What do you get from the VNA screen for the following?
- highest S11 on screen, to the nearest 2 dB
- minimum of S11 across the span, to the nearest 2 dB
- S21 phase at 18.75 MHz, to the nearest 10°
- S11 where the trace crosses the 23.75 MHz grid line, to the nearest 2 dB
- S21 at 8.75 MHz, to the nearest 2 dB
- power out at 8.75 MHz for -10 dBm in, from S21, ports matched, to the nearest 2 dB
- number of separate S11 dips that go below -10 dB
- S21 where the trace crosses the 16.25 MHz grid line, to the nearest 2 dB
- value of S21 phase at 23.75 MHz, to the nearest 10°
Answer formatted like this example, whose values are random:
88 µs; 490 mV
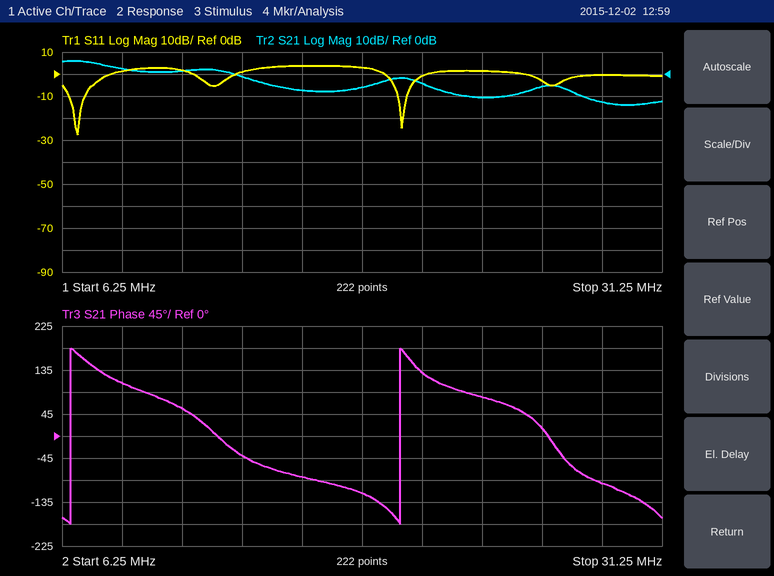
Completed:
4 dB; -28 dB; -120°; 2 dB; 2 dB; -8 dBm; 2; -8 dB; 80°
